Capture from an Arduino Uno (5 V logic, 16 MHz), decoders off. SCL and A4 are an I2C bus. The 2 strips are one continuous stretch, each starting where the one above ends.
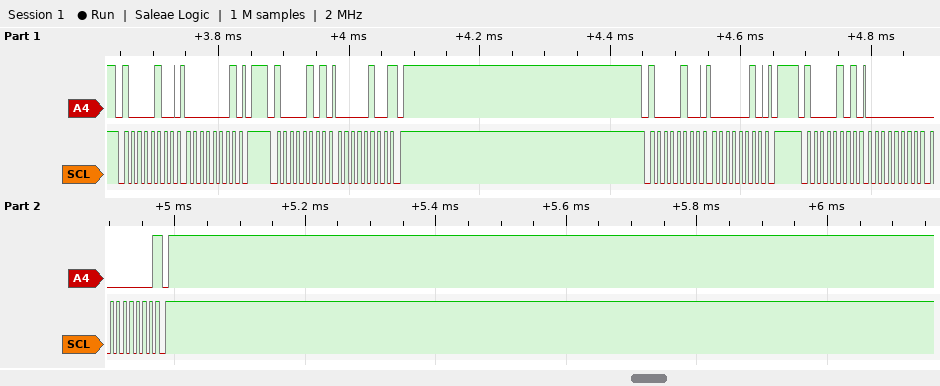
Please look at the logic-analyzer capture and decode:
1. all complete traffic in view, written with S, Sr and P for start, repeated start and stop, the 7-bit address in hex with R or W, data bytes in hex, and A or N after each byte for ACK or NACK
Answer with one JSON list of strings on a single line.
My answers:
["S 42W A 01 A P S 42R A 04 N P S 42W A 02 A P S 42R A 00 A 00 N P"]
